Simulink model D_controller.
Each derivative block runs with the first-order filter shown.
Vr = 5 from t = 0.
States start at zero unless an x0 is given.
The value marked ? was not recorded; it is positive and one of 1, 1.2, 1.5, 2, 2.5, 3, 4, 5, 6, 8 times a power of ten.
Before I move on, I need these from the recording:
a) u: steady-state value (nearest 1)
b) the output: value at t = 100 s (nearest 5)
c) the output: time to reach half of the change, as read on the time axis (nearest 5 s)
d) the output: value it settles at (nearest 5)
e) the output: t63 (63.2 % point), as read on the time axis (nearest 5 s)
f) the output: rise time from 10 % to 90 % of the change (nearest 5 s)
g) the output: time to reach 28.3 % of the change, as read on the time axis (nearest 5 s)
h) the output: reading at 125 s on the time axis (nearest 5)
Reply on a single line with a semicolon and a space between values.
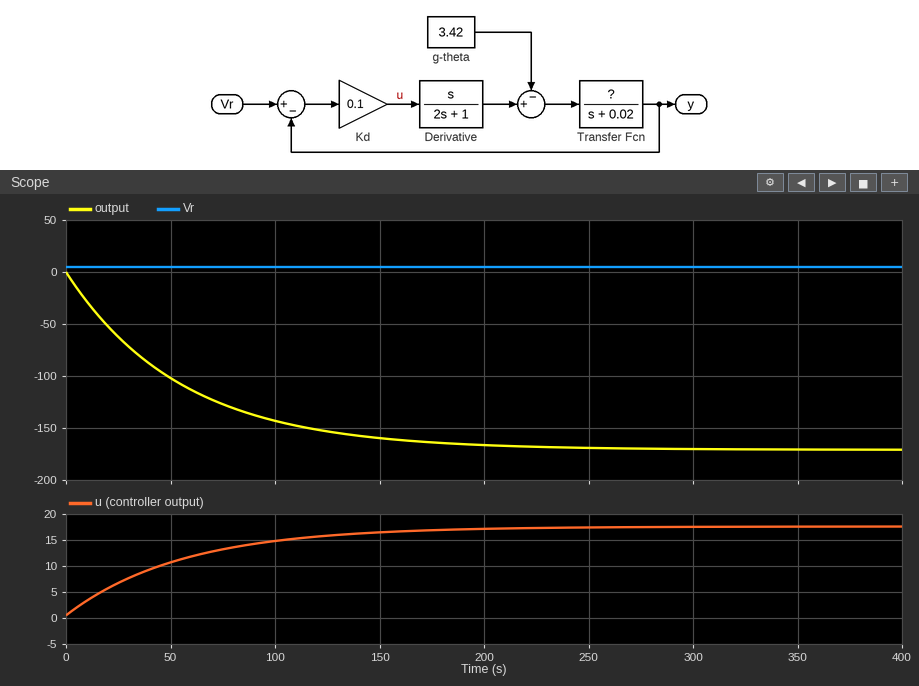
18; -145; 40 s; -170; 55 s; 120 s; 20 s; -155
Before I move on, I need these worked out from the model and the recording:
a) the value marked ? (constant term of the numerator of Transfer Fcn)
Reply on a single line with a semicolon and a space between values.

1
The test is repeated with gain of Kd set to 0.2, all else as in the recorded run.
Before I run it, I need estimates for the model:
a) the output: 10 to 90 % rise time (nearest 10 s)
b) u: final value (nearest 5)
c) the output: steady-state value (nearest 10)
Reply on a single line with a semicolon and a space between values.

130 s; 35; -170
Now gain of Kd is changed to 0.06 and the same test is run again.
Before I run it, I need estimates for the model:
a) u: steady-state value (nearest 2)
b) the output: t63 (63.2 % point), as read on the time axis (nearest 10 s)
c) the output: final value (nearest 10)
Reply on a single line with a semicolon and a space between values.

10; 50 s; -170
